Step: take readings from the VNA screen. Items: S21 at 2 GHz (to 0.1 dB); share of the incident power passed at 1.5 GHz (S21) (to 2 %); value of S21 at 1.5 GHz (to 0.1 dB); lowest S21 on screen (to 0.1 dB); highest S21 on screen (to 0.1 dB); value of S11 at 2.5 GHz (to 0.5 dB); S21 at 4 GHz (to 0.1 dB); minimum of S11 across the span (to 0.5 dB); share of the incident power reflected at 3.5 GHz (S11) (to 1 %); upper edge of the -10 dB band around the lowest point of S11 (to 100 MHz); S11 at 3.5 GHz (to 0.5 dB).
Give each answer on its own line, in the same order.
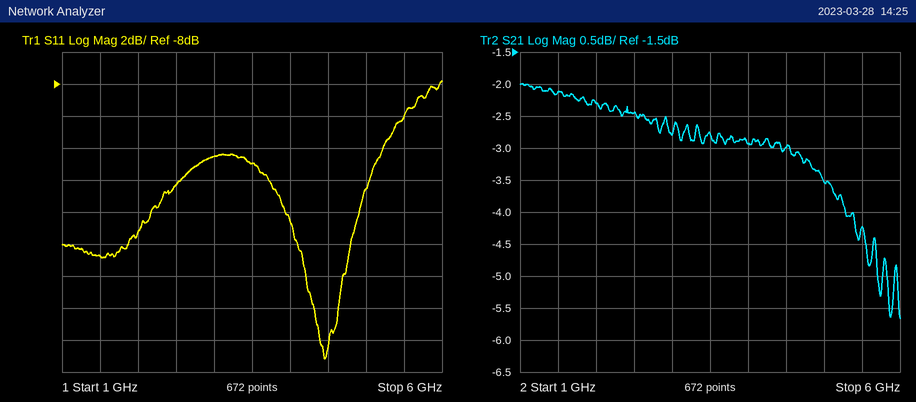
-2.3 dB
62 %
-2.1 dB
-5.7 dB
-2.0 dB
-14.5 dB
-2.9 dB
-25.0 dB
5 %
5.5 GHz
-13.0 dB
